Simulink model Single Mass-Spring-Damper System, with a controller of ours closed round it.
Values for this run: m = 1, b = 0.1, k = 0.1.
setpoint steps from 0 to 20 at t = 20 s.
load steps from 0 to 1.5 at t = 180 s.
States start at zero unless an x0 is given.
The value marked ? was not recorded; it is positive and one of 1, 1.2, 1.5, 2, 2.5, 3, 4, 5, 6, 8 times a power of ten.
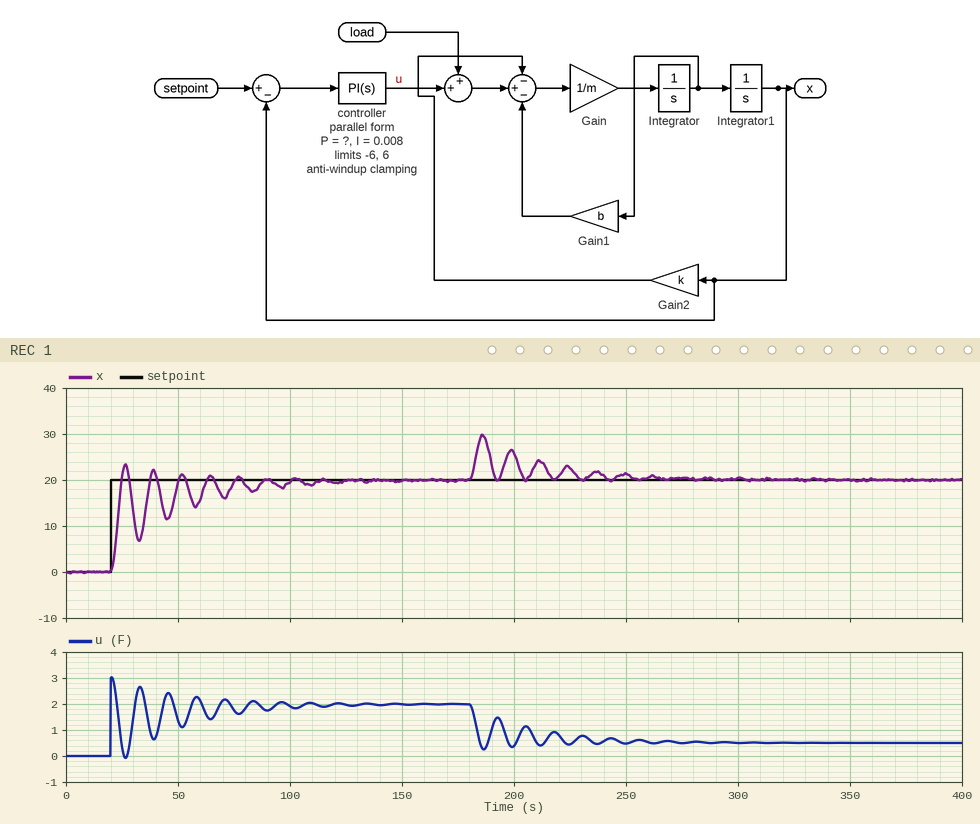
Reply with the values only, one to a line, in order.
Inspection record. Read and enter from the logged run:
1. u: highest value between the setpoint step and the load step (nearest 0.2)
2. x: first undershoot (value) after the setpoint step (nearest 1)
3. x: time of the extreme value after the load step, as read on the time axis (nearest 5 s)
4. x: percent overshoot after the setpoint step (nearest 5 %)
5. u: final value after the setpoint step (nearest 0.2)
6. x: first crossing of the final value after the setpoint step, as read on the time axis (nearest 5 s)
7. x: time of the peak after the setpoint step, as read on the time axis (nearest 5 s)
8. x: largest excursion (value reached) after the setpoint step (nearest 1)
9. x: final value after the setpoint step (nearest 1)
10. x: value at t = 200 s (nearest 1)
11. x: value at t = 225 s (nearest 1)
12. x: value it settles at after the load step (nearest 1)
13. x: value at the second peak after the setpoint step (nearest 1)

3.0
7
185 s
15 %
2.0
25 s
25 s
23
20
26
23
20
22
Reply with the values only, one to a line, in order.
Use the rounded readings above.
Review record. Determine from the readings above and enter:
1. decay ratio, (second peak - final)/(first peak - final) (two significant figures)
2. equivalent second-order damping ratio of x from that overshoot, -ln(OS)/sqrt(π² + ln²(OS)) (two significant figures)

0.67
0.52
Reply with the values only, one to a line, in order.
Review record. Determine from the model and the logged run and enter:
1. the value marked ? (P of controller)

0.15
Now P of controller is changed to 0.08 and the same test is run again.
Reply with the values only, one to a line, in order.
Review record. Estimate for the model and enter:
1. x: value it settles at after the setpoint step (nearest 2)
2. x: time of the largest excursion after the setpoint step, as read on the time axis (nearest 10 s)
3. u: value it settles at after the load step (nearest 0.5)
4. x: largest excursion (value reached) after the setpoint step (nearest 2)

20
60 s
0.5
22
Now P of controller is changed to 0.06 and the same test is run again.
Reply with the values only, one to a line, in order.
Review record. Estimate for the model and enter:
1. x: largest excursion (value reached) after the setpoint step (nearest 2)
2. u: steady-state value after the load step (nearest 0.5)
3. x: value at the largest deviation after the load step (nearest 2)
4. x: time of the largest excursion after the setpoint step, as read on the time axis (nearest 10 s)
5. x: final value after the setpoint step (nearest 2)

22
0.5
34
60 s
20
